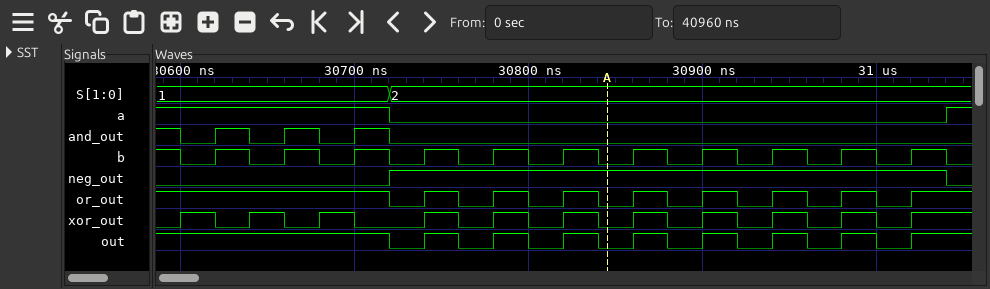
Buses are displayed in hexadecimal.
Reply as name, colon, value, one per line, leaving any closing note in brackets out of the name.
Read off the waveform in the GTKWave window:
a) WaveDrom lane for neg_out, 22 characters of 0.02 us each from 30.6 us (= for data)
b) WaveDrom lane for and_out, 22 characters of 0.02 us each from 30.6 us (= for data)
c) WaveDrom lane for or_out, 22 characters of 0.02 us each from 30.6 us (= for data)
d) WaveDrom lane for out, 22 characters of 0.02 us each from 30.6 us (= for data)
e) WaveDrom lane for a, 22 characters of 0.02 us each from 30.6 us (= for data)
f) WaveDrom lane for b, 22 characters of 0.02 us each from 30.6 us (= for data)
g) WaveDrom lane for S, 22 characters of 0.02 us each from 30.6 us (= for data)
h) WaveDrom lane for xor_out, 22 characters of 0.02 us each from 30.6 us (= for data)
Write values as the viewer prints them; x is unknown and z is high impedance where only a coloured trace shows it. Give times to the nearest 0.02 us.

WaveDrom lane for neg_out, 22 characters of 0.02 us each from 30.6 us: {name: 'neg_out', wave: '0.....1...............'}
WaveDrom lane for and_out, 22 characters of 0.02 us each from 30.6 us: {name: 'and_out', wave: '0101010...............'}
WaveDrom lane for or_out, 22 characters of 0.02 us each from 30.6 us: {name: 'or_out', wave: '1.....0101010101010101'}
WaveDrom lane for out, 22 characters of 0.02 us each from 30.6 us: {name: 'out', wave: '1.....0101010101010101'}
WaveDrom lane for a, 22 characters of 0.02 us each from 30.6 us: {name: 'a', wave: '1.....0...............'}
WaveDrom lane for b, 22 characters of 0.02 us each from 30.6 us: {name: 'b', wave: '0101010101010101010101'}
WaveDrom lane for S, 22 characters of 0.02 us each from 30.6 us: {name: 'S', wave: '=.....=...............', data: '1 2'}
WaveDrom lane for xor_out, 22 characters of 0.02 us each from 30.6 us: {name: 'xor_out', wave: '101010.101010101010101'}
